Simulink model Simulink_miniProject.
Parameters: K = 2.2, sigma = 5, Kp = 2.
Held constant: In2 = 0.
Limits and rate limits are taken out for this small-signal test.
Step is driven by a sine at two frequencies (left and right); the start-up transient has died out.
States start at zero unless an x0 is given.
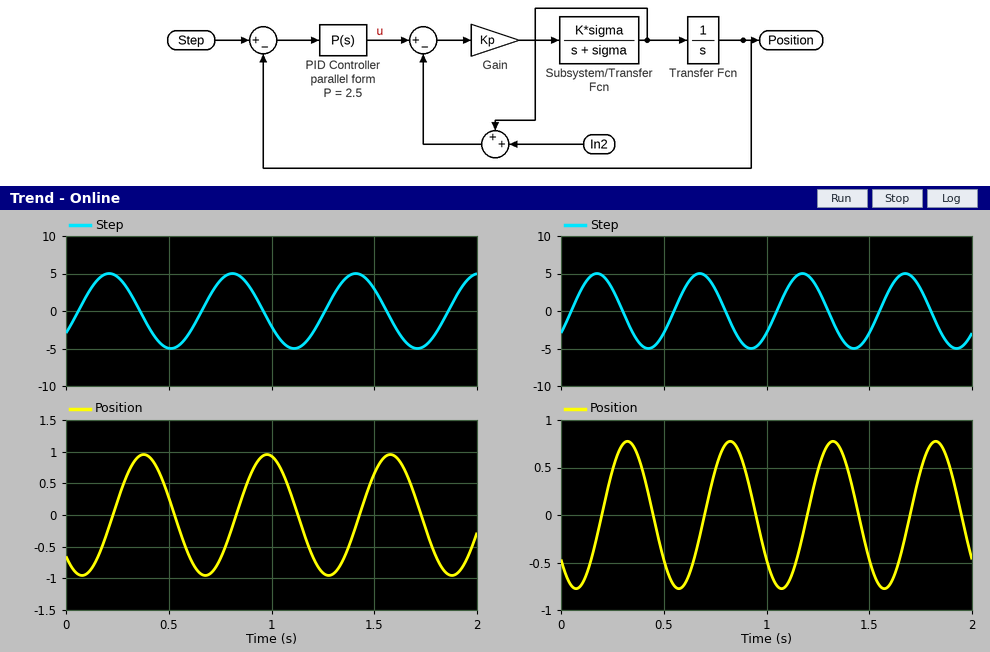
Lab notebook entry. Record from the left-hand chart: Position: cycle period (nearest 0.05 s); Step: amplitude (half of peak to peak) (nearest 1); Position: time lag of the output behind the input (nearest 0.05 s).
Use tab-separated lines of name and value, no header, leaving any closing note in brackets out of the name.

Position: cycle period	0.60 s
Step: amplitude (half of peak to peak)	5
Position: time lag of the output behind the input	0.15 s
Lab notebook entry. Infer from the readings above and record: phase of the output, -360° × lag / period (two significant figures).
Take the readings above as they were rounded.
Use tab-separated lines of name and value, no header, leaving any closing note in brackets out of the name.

phase of the output, -360° × lag / period	-90°
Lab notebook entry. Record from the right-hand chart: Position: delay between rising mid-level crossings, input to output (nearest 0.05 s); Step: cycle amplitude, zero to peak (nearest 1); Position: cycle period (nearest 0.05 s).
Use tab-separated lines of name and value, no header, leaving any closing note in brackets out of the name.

Position: delay between rising mid-level crossings, input to output	0.15 s
Step: cycle amplitude, zero to peak	5
Position: cycle period	0.50 s
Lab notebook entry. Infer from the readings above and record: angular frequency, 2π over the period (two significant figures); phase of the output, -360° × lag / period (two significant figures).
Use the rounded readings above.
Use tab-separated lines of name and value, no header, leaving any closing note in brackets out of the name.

angular frequency, 2π over the period	13 rad/s
phase of the output, -360° × lag / period	-110°
